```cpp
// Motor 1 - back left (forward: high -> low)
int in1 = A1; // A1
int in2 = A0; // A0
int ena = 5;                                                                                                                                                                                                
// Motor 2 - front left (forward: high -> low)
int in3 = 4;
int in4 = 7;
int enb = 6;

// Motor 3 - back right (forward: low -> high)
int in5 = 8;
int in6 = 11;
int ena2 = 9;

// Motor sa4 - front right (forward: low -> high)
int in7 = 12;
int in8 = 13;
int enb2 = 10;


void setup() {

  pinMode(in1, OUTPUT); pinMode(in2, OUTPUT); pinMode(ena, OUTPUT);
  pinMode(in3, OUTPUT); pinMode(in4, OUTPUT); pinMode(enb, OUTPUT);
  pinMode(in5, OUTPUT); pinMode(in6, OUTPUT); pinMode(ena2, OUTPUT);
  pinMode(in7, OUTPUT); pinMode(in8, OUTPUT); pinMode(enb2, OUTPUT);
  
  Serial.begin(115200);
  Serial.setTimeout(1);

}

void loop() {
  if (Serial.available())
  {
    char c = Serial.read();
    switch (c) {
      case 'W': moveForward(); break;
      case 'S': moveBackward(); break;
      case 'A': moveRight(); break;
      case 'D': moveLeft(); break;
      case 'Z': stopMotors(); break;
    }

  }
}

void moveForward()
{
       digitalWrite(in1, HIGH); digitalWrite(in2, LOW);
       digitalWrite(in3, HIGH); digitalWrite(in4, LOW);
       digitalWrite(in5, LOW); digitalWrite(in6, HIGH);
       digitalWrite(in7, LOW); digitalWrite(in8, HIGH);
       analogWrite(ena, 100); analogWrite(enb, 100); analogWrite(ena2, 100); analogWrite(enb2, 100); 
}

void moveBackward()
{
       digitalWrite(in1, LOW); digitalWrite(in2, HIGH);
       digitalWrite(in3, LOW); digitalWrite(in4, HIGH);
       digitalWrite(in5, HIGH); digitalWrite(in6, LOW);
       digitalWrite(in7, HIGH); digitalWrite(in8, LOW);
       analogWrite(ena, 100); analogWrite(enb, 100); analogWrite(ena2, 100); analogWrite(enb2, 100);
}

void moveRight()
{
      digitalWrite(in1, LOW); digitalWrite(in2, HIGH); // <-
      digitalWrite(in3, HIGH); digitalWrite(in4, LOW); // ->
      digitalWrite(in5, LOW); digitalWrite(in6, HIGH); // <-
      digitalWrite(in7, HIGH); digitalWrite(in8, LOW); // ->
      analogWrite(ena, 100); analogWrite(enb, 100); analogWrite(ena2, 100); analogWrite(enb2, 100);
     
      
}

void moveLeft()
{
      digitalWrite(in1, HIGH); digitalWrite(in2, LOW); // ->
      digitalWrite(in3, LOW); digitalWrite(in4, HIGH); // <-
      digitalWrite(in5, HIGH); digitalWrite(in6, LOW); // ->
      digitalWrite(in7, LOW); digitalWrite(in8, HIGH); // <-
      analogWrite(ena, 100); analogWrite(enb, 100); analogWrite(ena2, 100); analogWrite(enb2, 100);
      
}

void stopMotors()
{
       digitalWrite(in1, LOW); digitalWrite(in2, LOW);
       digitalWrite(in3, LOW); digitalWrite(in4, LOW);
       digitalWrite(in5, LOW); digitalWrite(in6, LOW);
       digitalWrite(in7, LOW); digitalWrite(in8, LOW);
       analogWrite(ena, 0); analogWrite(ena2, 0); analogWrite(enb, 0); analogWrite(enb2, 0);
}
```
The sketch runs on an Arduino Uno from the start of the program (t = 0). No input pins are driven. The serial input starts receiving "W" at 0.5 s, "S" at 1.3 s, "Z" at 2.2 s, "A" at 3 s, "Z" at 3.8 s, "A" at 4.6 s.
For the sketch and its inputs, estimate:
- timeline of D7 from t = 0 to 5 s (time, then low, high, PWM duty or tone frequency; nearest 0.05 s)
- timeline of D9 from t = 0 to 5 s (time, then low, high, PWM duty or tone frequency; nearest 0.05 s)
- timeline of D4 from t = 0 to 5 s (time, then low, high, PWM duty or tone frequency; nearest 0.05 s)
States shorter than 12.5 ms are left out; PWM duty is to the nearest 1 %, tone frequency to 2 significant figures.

0 s low; 1.3 s high; 2.2 s low
0 s low; 0.5 s PWM 39 %; 2.2 s low; 3 s PWM 39 %; 3.8 s low; 4.6 s PWM 39 %
0 s low; 0.5 s high; 1.3 s low; 3 s high; 3.8 s low; 4.6 s high
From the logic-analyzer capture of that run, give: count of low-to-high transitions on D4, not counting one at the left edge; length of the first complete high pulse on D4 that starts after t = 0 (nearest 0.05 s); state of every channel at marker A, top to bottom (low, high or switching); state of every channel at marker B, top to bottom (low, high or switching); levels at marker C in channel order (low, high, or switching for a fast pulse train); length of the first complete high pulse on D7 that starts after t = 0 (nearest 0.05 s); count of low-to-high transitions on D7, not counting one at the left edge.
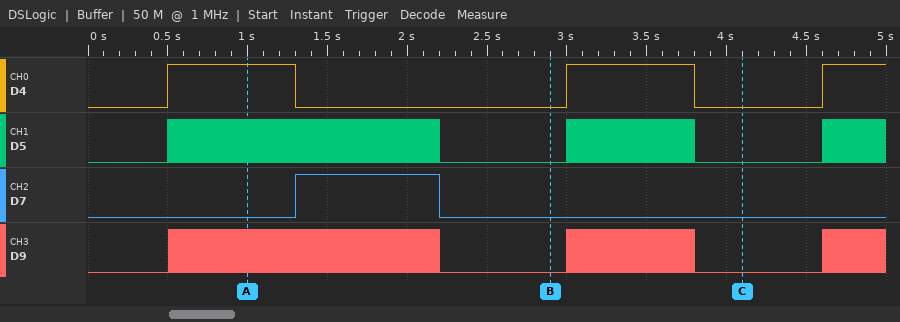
3
0.80 s
D4 high, D5 switching, D7 low, D9 switching
D4 low, D5 low, D7 low, D9 low
D4 low, D5 low, D7 low, D9 low
0.90 s
1
